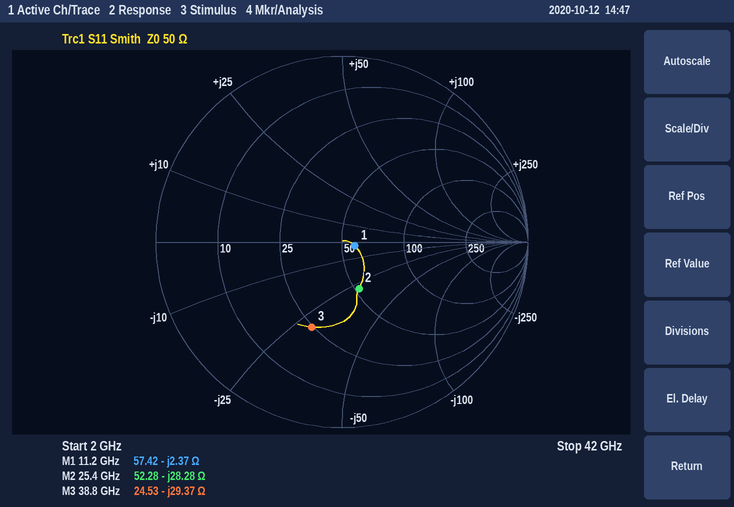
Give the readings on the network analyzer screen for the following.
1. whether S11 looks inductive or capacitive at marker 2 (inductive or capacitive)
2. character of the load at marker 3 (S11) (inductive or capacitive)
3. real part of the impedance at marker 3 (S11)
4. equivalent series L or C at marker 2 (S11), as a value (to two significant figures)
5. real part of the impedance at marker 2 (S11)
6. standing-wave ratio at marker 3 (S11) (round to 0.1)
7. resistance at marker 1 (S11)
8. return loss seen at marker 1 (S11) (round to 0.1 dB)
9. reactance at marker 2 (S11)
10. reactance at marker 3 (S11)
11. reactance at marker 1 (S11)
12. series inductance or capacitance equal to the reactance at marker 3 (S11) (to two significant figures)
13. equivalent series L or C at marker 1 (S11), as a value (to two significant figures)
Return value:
capacitive
capacitive
24.53 Ω
220 fF
52.28 Ω
2.9
57.42 Ω
22.8 dB
-28.28 Ω
-29.37 Ω
-2.37 Ω
140 fF
6.0 pF
